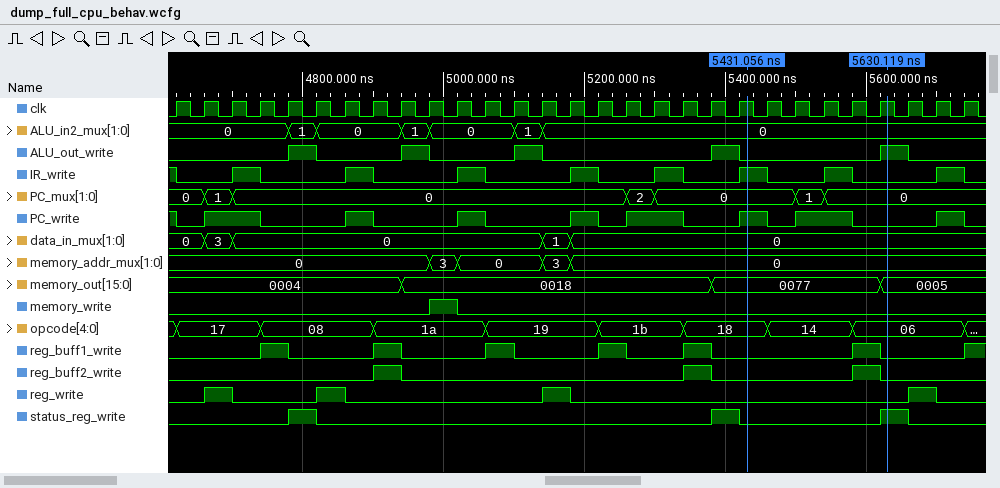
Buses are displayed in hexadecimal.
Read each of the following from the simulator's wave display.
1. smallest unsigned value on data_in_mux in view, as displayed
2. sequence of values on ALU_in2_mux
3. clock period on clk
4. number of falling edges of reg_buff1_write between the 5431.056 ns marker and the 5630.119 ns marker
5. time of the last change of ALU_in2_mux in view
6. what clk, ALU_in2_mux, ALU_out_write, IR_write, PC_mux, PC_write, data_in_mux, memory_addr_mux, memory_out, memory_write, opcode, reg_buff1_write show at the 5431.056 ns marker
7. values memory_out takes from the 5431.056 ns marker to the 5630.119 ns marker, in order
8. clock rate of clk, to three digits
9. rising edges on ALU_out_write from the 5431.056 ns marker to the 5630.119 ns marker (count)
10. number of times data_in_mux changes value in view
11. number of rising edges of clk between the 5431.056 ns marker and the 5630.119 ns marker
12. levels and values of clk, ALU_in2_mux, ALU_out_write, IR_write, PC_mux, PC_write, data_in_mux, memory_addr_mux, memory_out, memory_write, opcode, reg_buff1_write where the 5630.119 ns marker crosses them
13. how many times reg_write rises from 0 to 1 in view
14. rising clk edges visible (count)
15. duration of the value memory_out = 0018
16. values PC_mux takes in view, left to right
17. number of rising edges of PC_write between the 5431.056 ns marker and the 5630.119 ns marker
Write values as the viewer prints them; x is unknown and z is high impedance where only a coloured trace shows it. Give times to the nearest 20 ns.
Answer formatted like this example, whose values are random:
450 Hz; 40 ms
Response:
0; 0, 1, 0, 1, 0, 1, 0; 40 ns; 1; 5140 ns; clk=1, ALU_in2_mux=0, ALU_out_write=0, IR_write=1, PC_mux=0, PC_write=1, data_in_mux=0, memory_addr_mux=0, memory_out=0077, memory_write=0, opcode=18, reg_buff1_write=0; 0077, 0005; 25.0 MHz; 1; 4; 5; clk=1, ALU_in2_mux=0, ALU_out_write=1, IR_write=0, PC_mux=0, PC_write=0, data_in_mux=0, memory_addr_mux=0, memory_out=0005, memory_write=0, opcode=06, reg_buff1_write=0; 4; 29; 440 ns; 0, 1, 0, 2, 0, 1, 0; 1
